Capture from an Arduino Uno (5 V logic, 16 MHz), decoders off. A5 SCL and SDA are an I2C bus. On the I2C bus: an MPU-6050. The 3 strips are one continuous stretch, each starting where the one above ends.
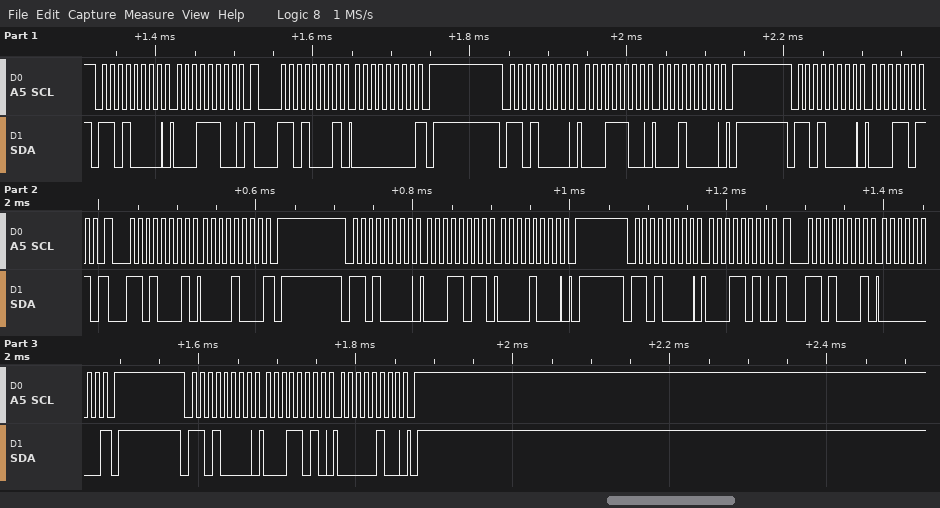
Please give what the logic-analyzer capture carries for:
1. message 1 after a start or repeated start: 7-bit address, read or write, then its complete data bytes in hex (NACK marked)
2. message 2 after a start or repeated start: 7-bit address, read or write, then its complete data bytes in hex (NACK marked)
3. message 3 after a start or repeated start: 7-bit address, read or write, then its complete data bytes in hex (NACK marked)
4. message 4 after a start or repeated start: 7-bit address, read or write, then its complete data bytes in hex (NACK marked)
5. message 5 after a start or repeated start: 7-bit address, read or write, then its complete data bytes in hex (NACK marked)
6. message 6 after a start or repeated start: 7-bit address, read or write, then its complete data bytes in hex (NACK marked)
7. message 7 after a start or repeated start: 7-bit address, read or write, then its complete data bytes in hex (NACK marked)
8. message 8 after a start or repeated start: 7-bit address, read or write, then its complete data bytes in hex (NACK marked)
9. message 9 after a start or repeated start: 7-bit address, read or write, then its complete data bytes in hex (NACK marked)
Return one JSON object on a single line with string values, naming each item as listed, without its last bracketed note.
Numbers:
{"message 1 after a start or repeated start: 7-bit address, read or write, then its complete data bytes in hex": "0x68 write: 1C", "message 2 after a start or repeated start: 7-bit address, read or write, then its complete data bytes in hex": "0x68 read: 00 NACK", "message 3 after a start or repeated start: 7-bit address, read or write, then its complete data bytes in hex": "0x68 write: 1C 10", "message 4 after a start or repeated start: 7-bit address, read or write, then its complete data bytes in hex": "0x68 write: 1B", "message 5 after a start or repeated start: 7-bit address, read or write, then its complete data bytes in hex": "0x68 read: 08 NACK", "message 6 after a start or repeated start: 7-bit address, read or write, then its complete data bytes in hex": "0x68 write: 1B 08", "message 7 after a start or repeated start: 7-bit address, read or write, then its complete data bytes in hex": "0x68 write: 1A", "message 8 after a start or repeated start: 7-bit address, read or write, then its complete data bytes in hex": "0x68 read: 00 NACK", "message 9 after a start or repeated start: 7-bit address, read or write, then its complete data bytes in hex": "0x68 write: 1A 04"}
